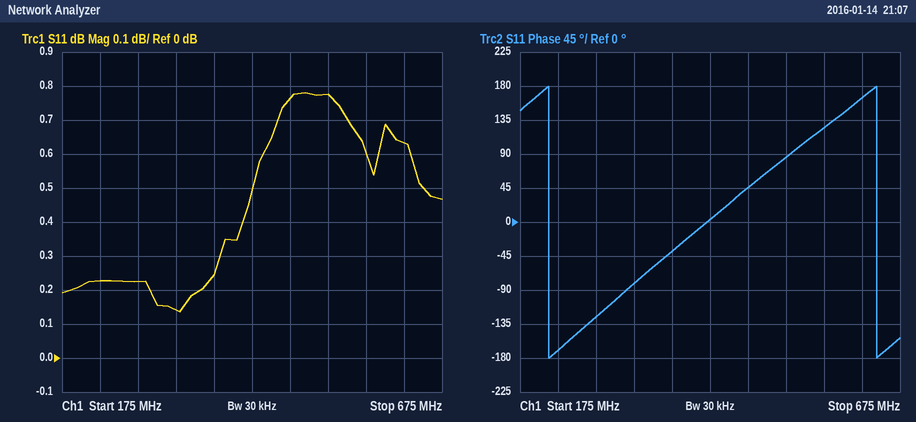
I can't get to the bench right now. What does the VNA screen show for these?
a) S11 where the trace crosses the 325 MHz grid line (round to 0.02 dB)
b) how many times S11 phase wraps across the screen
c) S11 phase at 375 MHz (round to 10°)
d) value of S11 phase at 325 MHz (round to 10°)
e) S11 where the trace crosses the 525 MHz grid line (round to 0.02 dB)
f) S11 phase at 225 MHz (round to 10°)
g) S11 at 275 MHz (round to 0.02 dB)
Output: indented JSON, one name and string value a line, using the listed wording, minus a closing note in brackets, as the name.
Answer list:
{
  "S11 where the trace crosses the 325 MHz grid line": "0.14 dB",
  "how many times S11 phase wraps across the screen": "2",
  "S11 phase at 375 MHz": "-40°",
  "value of S11 phase at 325 MHz": "-80°",
  "S11 where the trace crosses the 525 MHz grid line": "0.78 dB",
  "S11 phase at 225 MHz": "-170°",
  "S11 at 275 MHz": "0.22 dB"
}
